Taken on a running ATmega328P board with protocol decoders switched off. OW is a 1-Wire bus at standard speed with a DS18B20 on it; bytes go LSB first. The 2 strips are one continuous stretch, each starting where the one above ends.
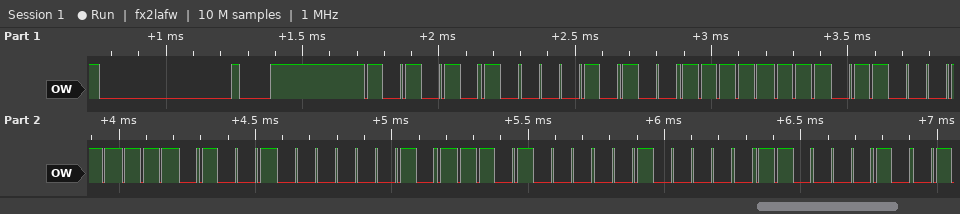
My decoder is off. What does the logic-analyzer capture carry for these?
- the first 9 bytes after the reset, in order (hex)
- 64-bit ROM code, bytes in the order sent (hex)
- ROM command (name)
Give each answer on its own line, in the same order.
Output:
55 28 FF C6 97 40 17 04 43
28 FF C6 97 40 17 04 43
Match ROM
